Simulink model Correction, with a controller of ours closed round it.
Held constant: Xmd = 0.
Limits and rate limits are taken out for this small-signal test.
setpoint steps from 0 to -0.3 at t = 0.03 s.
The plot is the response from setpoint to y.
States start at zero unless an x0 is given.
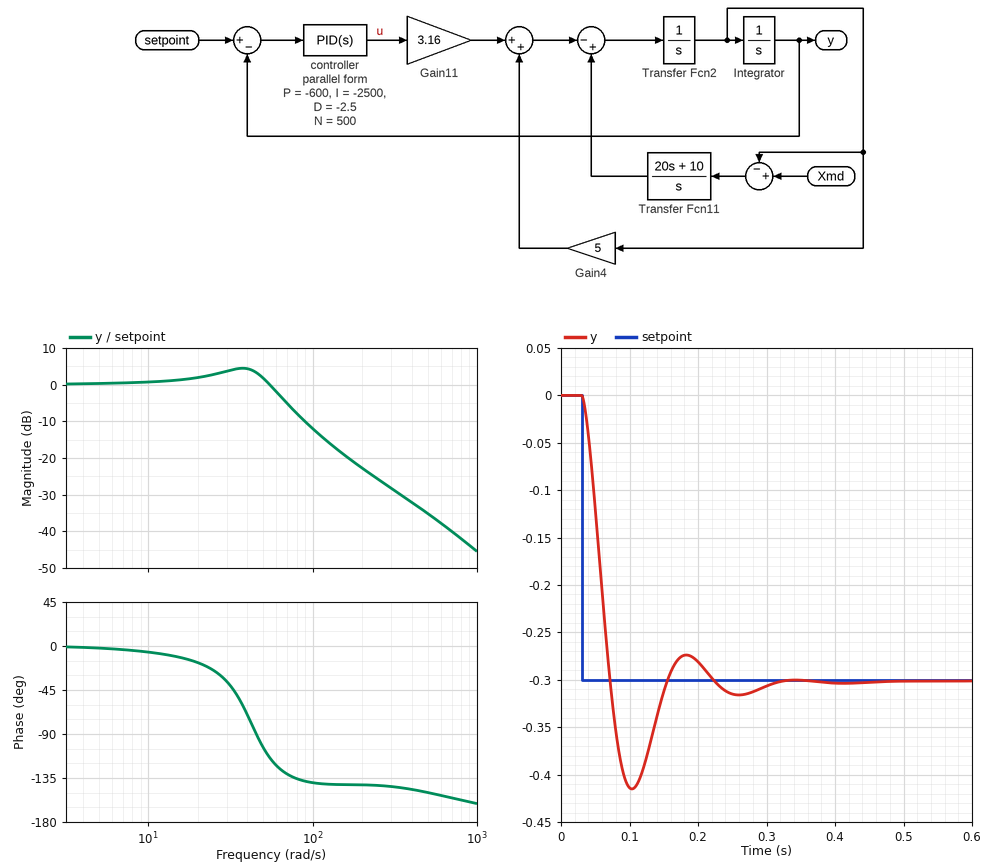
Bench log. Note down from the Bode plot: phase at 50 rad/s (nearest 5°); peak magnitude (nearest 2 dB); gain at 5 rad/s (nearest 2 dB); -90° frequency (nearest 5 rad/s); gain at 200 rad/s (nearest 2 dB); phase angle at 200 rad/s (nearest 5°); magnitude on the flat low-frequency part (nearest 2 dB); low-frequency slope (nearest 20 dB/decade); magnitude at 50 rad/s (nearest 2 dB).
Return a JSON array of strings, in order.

["-105°", "4 dB", "0 dB", "45 rad/s", "-22 dB", "-140°", "0 dB", "0 dB/decade", "2 dB"]
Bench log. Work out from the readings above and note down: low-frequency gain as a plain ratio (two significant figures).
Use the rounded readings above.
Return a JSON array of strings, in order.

["1.0"]
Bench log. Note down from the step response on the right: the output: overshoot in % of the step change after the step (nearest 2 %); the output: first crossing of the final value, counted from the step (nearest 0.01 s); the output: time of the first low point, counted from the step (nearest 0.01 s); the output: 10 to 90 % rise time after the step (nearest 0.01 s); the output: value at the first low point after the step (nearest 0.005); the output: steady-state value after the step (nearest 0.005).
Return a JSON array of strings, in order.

["38 %", "0.04 s", "0.07 s", "0.03 s", "-0.415", "-0.300"]
